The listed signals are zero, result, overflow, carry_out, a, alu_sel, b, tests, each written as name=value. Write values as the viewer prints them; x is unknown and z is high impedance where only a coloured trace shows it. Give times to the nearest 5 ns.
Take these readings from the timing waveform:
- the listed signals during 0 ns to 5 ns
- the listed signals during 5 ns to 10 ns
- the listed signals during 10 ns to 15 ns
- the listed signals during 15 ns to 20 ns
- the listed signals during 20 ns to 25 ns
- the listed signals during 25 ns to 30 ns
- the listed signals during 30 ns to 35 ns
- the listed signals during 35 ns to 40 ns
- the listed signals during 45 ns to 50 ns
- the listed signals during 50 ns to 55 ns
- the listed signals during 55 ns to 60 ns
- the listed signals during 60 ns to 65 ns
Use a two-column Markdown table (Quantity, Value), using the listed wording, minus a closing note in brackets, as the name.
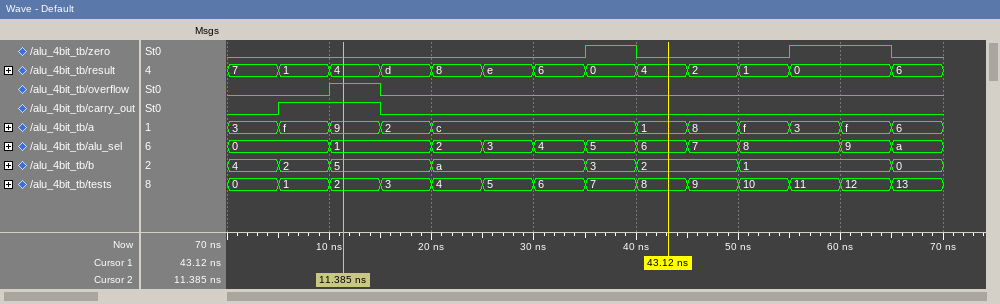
| Quantity | Value |
|---|---|
| the listed signals during 0 ns to 5 ns | zero=0, result=7, overflow=0, carry_out=0, a=3, alu_sel=0, b=4, tests=0 |
| the listed signals during 5 ns to 10 ns | zero=0, result=1, overflow=0, carry_out=1, a=f, alu_sel=0, b=2, tests=1 |
| the listed signals during 10 ns to 15 ns | zero=0, result=4, overflow=1, carry_out=1, a=9, alu_sel=1, b=5, tests=2 |
| the listed signals during 15 ns to 20 ns | zero=0, result=d, overflow=0, carry_out=0, a=2, alu_sel=1, b=5, tests=3 |
| the listed signals during 20 ns to 25 ns | zero=0, result=8, overflow=0, carry_out=0, a=c, alu_sel=2, b=a, tests=4 |
| the listed signals during 25 ns to 30 ns | zero=0, result=e, overflow=0, carry_out=0, a=c, alu_sel=3, b=a, tests=5 |
| the listed signals during 30 ns to 35 ns | zero=0, result=6, overflow=0, carry_out=0, a=c, alu_sel=4, b=a, tests=6 |
| the listed signals during 35 ns to 40 ns | zero=1, result=0, overflow=0, carry_out=0, a=c, alu_sel=5, b=3, tests=7 |
| the listed signals during 45 ns to 50 ns | zero=0, result=2, overflow=0, carry_out=0, a=8, alu_sel=7, b=2, tests=9 |
| the listed signals during 50 ns to 55 ns | zero=0, result=1, overflow=0, carry_out=0, a=f, alu_sel=8, b=1, tests=10 |
| the listed signals during 55 ns to 60 ns | zero=1, result=0, overflow=0, carry_out=0, a=3, alu_sel=8, b=1, tests=11 |
| the listed signals during 60 ns to 65 ns | zero=1, result=0, overflow=0, carry_out=0, a=f, alu_sel=9, b=1, tests=12 |
